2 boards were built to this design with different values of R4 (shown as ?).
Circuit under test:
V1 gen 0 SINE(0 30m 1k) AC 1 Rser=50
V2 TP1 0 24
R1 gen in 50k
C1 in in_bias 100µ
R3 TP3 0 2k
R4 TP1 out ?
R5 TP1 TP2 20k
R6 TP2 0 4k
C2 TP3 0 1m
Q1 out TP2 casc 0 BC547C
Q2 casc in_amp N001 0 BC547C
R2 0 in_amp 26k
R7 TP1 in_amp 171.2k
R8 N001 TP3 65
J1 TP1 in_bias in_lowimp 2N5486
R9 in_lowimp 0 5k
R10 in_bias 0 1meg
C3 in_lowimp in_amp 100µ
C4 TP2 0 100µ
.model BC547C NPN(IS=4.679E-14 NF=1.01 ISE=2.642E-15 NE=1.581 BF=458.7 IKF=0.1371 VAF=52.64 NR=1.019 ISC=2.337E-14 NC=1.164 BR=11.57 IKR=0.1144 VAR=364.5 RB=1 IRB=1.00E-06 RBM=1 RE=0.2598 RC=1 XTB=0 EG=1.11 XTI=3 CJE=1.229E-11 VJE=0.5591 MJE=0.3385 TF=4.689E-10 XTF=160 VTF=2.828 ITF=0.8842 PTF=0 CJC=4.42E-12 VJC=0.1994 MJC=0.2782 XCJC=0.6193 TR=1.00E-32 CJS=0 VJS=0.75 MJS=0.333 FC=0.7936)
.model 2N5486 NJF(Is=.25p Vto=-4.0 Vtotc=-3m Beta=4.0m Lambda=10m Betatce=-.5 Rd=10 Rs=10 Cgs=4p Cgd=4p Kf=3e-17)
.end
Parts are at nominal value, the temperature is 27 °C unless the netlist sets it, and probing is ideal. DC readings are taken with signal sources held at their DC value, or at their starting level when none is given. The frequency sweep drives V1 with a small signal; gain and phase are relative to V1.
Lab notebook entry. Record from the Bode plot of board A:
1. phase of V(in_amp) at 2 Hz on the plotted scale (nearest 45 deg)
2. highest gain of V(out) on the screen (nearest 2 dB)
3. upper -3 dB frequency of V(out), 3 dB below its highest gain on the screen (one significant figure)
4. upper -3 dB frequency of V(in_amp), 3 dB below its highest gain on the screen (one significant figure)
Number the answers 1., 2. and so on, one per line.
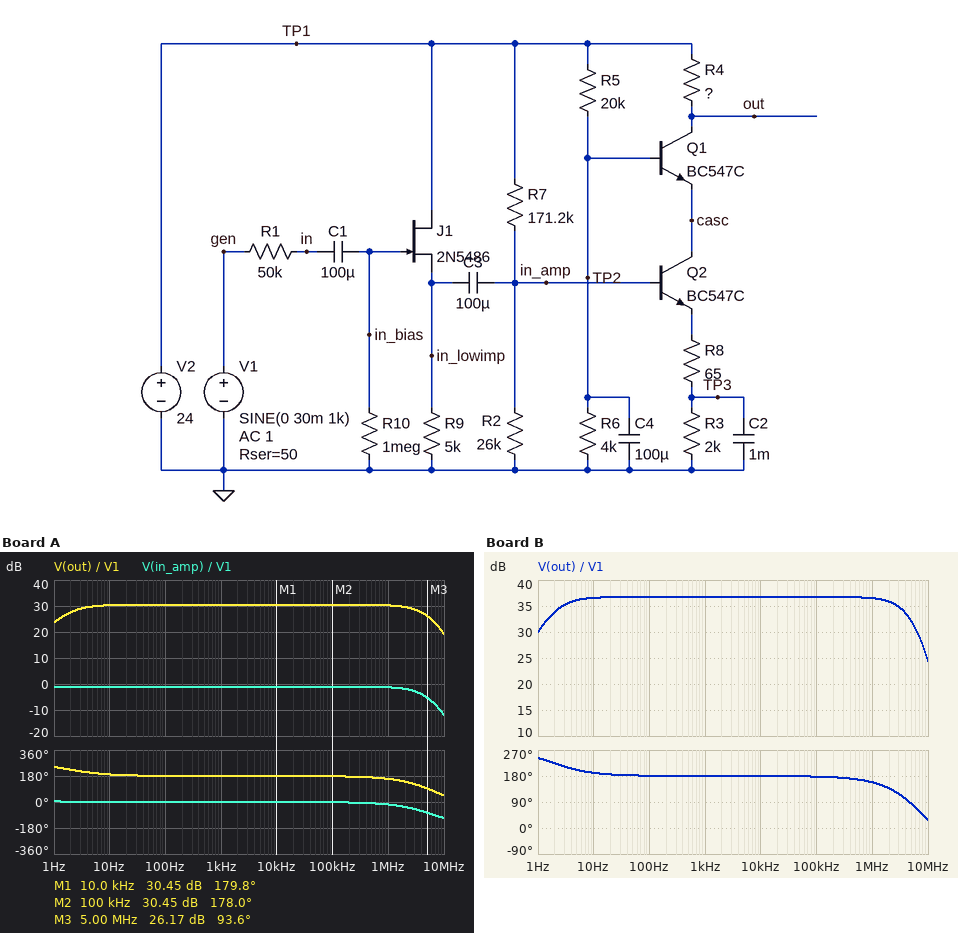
1. 0 deg
2. 30 dB
3. 4 MHz
4. 4 MHz
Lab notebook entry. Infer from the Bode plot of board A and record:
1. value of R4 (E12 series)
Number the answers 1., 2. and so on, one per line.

1. 3.3 kΩ
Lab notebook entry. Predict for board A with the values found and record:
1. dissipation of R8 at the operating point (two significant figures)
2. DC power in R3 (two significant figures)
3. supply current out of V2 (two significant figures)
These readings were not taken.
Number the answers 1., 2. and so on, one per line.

1. 94 µW
2. 2.9 mW
3. 3.0 mA
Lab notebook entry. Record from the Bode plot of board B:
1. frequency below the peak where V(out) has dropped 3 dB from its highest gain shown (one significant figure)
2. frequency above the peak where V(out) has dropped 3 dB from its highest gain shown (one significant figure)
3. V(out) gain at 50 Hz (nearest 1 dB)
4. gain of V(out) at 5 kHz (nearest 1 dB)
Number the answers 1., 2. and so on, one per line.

1. 2 Hz
2. 4 MHz
3. 37 dB
4. 37 dB
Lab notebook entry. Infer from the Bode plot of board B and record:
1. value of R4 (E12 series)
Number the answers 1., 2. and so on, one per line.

1. 6.8 kΩ
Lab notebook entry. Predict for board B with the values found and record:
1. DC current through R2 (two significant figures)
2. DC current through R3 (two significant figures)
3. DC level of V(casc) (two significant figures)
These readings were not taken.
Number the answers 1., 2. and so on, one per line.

1. 120 µA
2. 1.2 mA
3. 3.4 V
